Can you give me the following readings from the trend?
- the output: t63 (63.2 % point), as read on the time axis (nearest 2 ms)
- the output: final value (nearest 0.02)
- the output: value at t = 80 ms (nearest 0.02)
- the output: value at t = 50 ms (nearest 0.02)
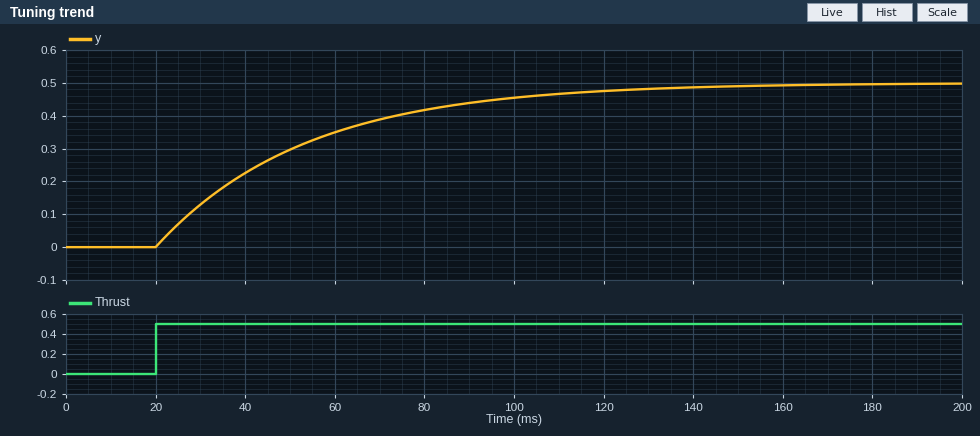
54 ms
0.50
0.42
0.30
